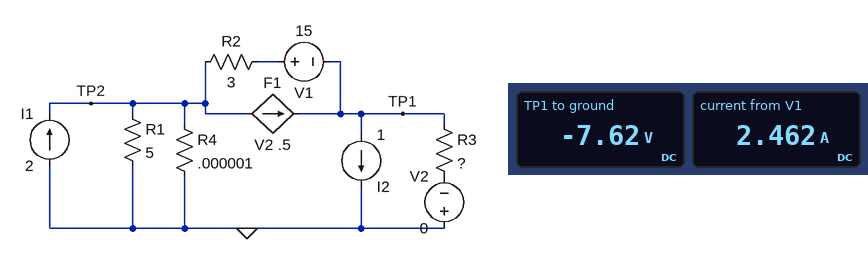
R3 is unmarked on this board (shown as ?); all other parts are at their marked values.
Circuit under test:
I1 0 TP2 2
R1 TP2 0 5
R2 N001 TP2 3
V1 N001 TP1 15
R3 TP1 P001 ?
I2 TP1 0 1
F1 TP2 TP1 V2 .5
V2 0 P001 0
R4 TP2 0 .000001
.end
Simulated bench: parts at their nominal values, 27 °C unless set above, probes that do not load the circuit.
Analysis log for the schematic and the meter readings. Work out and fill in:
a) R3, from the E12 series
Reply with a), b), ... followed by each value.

a) 3.3 Ω
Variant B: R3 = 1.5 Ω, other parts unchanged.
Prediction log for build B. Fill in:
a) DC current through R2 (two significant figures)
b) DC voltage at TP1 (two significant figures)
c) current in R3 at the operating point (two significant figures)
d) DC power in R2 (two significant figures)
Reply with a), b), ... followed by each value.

a) 3.5 A
b) -4.5 V
c) 3.0 A
d) 37 W
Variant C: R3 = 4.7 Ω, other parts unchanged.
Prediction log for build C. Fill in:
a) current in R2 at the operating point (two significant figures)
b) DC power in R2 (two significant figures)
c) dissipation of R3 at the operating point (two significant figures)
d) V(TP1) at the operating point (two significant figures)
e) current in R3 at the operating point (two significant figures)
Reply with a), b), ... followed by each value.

a) 1.9 A
b) 11 W
c) 18 W
d) -9.2 V
e) 2.0 A
